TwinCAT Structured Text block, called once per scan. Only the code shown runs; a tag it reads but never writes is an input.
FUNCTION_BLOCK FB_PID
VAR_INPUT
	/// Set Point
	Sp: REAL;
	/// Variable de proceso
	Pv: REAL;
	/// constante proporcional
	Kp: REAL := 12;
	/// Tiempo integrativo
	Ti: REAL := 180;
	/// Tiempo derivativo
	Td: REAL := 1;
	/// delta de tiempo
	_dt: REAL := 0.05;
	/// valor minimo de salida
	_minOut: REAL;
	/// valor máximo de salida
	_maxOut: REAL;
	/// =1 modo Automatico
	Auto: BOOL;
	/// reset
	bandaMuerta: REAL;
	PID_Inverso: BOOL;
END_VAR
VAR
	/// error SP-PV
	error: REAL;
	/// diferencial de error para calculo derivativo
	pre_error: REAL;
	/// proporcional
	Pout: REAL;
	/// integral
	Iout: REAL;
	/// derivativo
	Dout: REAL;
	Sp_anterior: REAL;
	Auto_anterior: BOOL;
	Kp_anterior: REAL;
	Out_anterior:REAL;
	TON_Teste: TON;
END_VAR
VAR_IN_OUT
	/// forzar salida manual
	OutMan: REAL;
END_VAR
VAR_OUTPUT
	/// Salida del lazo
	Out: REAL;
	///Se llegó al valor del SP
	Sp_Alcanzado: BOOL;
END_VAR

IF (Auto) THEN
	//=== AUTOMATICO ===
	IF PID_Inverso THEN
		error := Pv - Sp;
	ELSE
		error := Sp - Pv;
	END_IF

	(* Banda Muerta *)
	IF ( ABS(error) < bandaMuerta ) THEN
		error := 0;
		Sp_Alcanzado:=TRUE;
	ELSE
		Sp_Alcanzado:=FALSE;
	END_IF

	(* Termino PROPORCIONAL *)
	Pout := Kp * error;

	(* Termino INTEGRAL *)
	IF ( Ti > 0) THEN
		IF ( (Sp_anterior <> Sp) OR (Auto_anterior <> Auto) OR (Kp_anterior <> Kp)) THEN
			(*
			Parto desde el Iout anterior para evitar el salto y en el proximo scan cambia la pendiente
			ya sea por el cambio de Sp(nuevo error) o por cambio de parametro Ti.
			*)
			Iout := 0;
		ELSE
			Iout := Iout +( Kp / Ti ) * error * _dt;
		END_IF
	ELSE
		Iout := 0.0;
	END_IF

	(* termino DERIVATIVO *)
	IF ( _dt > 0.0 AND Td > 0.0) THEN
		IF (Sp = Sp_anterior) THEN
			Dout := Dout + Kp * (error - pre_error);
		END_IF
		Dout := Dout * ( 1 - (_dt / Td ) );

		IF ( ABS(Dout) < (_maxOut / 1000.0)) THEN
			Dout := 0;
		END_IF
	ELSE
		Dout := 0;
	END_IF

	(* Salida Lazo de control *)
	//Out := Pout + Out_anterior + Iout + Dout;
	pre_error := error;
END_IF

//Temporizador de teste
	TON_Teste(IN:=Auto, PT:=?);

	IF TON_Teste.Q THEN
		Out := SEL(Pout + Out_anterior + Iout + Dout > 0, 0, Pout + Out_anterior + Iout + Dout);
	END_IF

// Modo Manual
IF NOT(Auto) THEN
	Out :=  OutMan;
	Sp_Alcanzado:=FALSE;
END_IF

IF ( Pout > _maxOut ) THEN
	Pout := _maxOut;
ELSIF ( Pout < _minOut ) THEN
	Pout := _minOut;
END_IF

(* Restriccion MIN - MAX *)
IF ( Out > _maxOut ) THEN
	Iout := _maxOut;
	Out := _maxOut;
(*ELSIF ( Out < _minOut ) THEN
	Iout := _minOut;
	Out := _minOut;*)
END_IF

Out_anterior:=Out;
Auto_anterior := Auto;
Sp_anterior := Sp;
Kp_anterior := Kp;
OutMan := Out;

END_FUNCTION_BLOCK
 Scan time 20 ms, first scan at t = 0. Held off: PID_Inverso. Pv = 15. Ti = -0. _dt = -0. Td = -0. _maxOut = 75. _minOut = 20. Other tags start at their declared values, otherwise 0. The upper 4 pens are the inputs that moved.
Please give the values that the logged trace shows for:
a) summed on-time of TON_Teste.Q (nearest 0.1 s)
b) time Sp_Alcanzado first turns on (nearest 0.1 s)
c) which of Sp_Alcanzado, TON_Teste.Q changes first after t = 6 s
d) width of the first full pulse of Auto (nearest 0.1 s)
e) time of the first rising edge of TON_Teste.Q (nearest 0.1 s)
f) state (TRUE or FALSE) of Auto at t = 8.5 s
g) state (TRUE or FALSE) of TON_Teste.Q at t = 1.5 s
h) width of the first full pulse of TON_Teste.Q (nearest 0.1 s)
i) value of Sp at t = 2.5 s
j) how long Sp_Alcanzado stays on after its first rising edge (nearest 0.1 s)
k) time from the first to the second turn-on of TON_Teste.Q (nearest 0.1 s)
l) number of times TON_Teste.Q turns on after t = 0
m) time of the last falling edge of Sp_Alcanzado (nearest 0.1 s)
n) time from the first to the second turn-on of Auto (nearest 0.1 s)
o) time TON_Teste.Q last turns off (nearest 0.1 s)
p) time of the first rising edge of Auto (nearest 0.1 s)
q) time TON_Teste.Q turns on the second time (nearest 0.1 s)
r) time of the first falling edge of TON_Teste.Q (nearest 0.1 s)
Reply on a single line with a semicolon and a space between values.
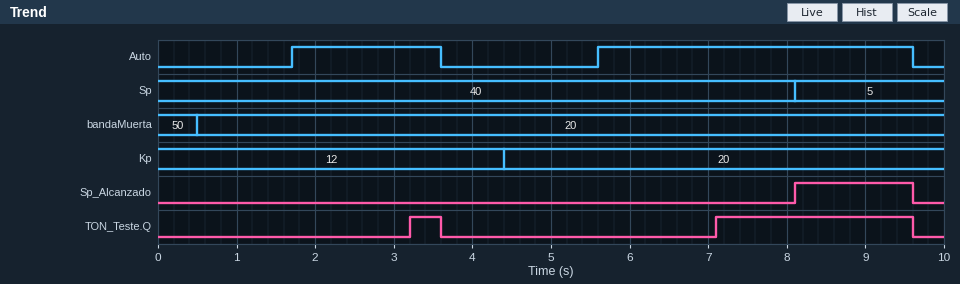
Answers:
2.9 s; 8.1 s; TON_Teste.Q; 1.9 s; 3.2 s; TRUE; FALSE; 0.4 s; 40; 1.5 s; 3.9 s; 2; 9.6 s; 3.9 s; 9.6 s; 1.7 s; 7.1 s; 3.6 s
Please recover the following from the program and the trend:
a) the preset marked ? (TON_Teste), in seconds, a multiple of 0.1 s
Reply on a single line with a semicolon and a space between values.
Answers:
1.5 s
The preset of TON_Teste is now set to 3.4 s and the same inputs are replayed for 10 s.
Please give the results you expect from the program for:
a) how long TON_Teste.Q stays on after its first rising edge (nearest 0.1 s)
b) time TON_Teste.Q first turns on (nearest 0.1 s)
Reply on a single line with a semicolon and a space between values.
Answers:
0.6 s; 9.0 s
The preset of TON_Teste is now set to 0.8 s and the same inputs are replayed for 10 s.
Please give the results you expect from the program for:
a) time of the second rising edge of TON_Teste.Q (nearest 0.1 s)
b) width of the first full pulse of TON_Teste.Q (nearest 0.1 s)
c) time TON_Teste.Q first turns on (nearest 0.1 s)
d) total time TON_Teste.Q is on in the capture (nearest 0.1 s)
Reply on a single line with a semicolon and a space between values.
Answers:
6.4 s; 1.1 s; 2.5 s; 4.3 s
